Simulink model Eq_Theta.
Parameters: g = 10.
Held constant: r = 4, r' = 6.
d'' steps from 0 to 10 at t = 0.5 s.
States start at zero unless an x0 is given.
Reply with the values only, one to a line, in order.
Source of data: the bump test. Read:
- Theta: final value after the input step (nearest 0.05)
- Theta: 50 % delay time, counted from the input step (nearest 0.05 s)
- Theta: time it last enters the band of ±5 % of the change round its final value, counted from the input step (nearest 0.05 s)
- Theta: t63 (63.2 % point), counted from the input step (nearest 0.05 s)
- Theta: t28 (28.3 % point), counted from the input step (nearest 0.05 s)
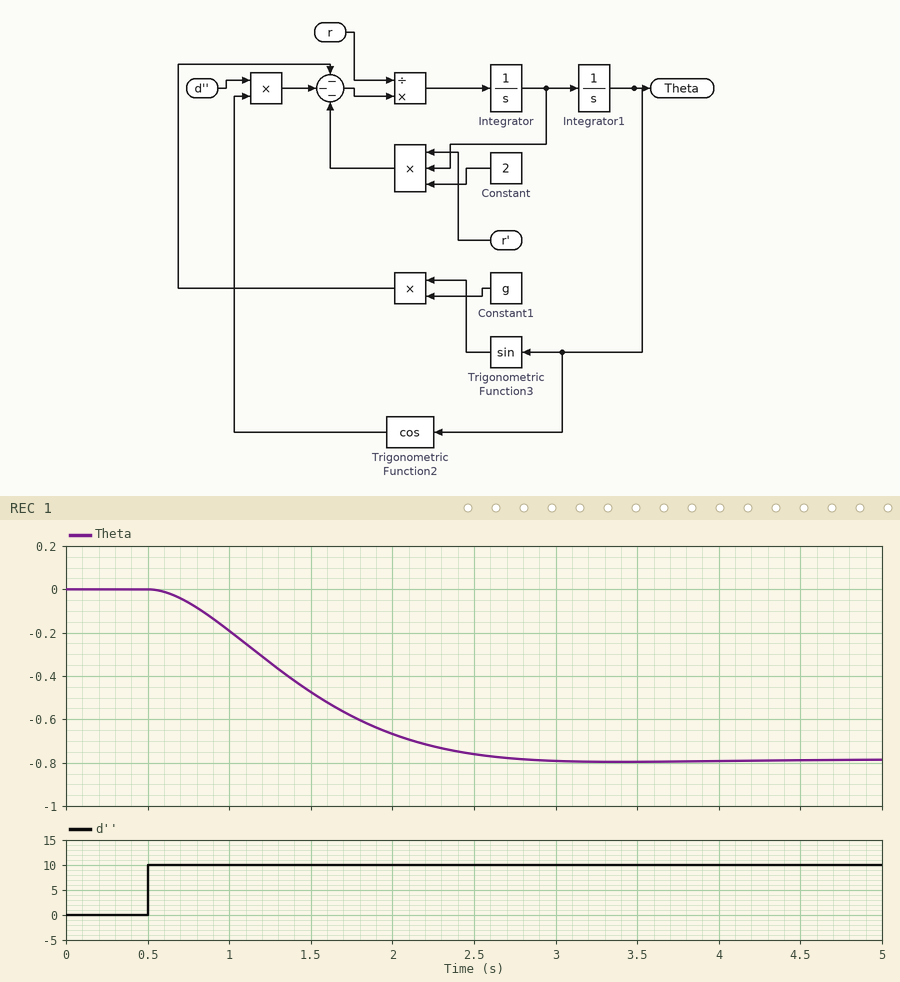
-0.80
0.85 s
1.90 s
1.05 s
0.55 s
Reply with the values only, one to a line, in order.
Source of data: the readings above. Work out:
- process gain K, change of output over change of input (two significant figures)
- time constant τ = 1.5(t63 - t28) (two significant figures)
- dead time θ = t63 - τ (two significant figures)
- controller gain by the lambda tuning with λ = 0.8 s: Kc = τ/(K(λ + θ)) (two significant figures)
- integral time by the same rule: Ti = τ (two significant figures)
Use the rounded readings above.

-0.080
0.75 s
0.30 s
-8.5
0.75 s
